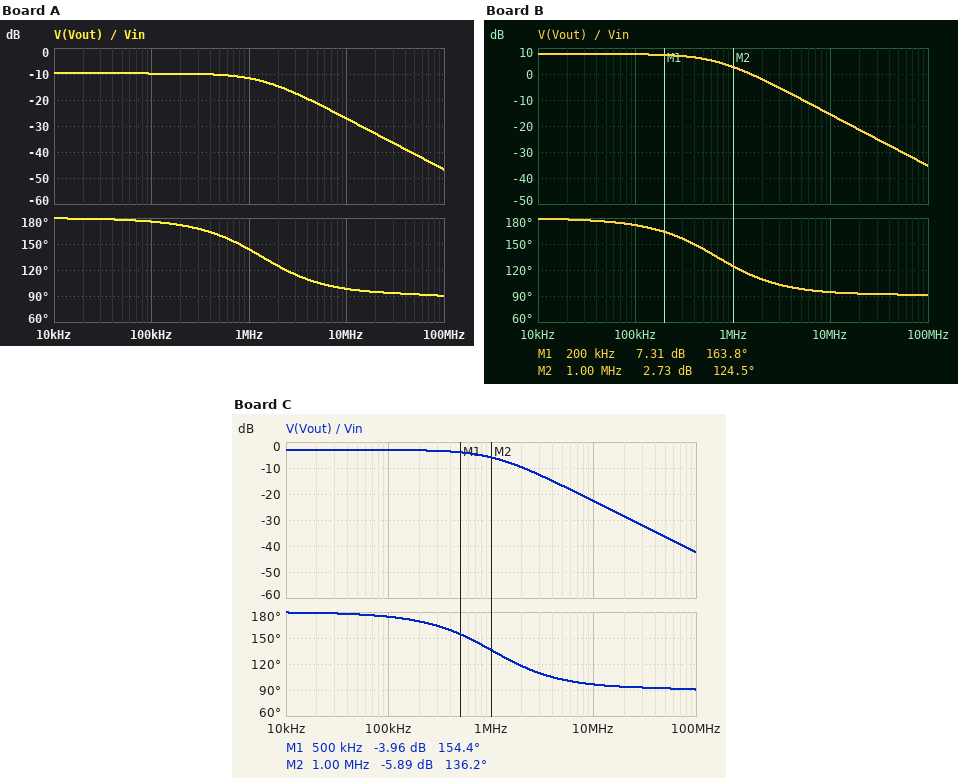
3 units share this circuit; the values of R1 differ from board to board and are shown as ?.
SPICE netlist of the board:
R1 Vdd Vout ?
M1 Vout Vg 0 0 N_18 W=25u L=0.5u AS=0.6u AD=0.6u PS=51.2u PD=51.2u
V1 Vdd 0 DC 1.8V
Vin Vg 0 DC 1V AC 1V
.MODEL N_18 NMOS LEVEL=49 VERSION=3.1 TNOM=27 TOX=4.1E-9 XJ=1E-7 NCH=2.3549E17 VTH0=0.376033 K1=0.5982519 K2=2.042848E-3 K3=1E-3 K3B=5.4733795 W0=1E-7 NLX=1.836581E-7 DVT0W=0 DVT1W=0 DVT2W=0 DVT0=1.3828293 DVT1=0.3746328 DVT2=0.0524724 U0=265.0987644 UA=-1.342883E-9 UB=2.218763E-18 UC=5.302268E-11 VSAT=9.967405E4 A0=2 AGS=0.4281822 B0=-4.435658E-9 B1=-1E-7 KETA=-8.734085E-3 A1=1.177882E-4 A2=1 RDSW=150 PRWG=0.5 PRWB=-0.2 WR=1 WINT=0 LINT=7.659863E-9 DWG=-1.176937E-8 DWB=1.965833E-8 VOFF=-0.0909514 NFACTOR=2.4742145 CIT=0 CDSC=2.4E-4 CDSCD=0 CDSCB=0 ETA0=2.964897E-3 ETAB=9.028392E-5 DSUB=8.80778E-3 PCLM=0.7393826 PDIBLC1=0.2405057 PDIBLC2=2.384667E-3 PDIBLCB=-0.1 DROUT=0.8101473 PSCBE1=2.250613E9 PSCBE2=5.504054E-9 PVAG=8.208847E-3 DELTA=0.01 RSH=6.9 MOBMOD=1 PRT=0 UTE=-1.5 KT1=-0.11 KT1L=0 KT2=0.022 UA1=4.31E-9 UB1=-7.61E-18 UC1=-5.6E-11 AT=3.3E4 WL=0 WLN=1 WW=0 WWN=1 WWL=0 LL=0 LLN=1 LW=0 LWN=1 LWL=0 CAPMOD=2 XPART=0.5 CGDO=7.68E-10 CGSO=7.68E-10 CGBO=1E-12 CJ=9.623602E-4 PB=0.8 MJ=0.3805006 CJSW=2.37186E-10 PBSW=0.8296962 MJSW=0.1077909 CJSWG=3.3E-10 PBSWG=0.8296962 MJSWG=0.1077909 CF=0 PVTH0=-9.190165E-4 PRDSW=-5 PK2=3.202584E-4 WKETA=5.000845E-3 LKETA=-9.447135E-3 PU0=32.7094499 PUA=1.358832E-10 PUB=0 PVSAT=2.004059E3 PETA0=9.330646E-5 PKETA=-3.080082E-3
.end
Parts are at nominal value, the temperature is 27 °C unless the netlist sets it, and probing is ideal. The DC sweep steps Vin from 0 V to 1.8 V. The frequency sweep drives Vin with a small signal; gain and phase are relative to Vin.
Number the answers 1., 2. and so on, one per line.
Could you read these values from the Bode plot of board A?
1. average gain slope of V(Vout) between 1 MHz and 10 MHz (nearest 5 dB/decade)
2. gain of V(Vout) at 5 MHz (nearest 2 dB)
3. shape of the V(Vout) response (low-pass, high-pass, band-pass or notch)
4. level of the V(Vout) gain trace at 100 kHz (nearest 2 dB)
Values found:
1. -15 dB/decade
2. -22 dB
3. low-pass
4. -10 dB
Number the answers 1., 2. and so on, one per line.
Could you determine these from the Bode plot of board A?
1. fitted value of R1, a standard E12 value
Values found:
1. 2.2 kΩ
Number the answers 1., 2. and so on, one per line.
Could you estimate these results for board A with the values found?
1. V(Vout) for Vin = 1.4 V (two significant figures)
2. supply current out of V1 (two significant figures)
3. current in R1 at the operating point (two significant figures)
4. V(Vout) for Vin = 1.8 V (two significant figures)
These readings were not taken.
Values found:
1. 85 mV
2. 750 µA
3. 750 µA
4. 69 mV
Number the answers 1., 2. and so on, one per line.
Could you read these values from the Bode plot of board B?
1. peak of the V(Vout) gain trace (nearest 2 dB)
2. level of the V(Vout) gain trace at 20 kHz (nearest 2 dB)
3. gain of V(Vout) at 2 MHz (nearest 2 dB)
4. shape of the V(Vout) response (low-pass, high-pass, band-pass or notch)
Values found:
1. 8 dB
2. 8 dB
3. -2 dB
4. low-pass
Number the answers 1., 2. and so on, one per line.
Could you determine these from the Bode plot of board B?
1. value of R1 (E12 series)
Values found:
1. 560 Ω
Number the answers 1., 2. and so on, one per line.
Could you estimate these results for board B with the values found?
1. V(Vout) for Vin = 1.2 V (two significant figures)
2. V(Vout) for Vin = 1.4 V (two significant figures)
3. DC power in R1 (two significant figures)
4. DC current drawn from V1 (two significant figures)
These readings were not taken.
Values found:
1. 530 mV
2. 360 mV
3. 1.1 mW
4. 1.4 mA
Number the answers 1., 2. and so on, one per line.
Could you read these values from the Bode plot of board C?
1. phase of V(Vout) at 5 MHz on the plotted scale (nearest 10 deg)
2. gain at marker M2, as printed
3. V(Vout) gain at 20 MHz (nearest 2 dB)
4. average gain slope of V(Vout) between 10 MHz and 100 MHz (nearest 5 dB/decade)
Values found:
1. 100 deg
2. -5.89 dB
3. -28 dB
4. -20 dB/decade
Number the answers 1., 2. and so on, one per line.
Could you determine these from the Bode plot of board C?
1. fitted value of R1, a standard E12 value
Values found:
1. 1.5 kΩ
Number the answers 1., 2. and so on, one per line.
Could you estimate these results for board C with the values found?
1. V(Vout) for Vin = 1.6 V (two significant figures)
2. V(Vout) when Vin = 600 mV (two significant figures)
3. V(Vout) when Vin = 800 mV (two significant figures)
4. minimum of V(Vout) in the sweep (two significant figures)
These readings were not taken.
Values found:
1. 110 mV
2. 1.6 V
3. 880 mV
4. 100 mV
